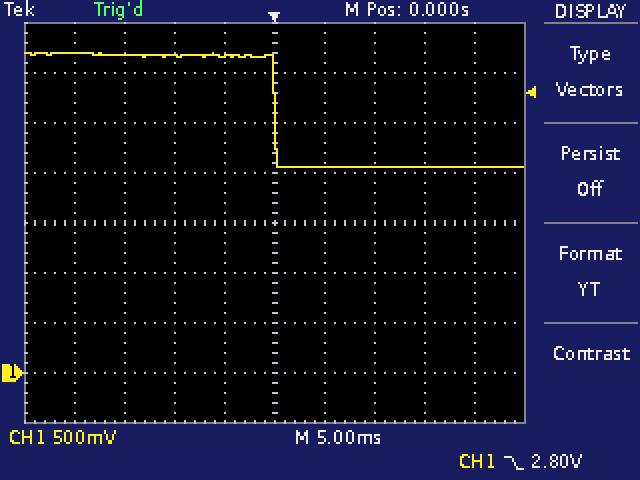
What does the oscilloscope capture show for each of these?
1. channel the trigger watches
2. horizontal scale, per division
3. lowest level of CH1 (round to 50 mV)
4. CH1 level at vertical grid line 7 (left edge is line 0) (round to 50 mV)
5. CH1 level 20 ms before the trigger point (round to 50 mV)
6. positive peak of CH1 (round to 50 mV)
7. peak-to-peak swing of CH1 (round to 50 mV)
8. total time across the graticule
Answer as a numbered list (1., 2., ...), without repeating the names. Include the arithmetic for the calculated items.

1. CH1
2. 5 ms
3. 2.05 V
4. 2.05 V
5. 3.20 V
6. 3.20 V
7. 3.20 V − (2.05 V) = 1.15 V
8. 50 ms
